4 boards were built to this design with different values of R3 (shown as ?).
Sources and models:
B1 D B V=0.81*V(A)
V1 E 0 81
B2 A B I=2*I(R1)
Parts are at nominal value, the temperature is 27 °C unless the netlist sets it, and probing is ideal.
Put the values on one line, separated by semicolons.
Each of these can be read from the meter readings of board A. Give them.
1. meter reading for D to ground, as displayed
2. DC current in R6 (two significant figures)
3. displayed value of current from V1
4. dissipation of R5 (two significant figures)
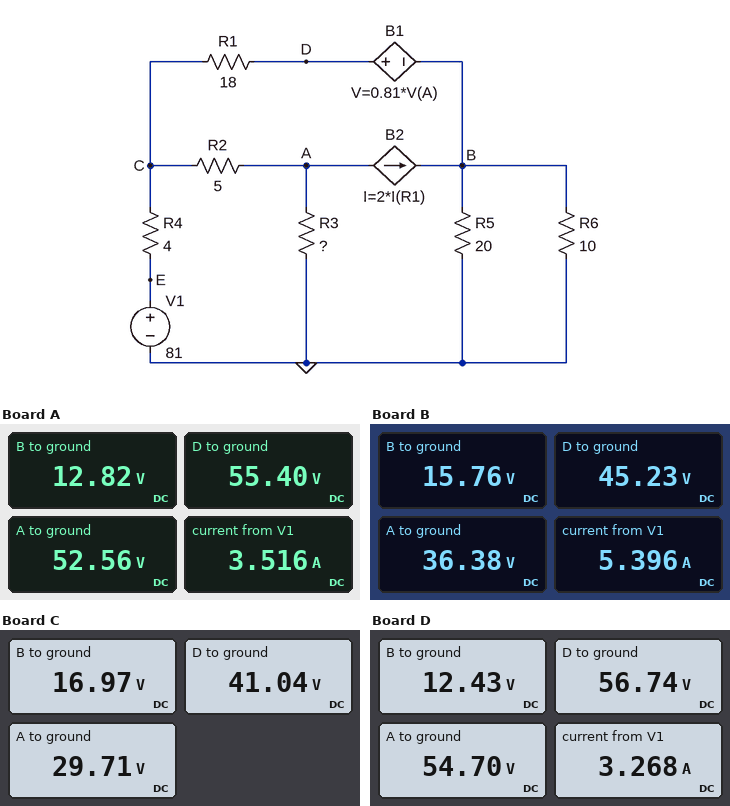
55.40 V; 1.3 A; 3.516 A; 8.2 W
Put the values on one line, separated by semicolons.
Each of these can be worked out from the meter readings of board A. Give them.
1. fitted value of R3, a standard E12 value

33 Ω
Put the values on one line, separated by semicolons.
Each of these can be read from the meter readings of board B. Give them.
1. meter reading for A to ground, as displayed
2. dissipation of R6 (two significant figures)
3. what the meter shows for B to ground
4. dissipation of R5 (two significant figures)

36.38 V; 25 W; 15.76 V; 12 W
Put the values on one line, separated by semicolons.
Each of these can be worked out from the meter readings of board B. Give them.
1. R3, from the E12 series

12 Ω
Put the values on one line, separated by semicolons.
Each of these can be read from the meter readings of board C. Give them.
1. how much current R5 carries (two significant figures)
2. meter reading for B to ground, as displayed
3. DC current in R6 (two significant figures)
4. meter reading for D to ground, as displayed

850 mA; 16.97 V; 1.7 A; 41.04 V
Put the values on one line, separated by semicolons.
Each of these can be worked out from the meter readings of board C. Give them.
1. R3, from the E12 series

8.2 Ω
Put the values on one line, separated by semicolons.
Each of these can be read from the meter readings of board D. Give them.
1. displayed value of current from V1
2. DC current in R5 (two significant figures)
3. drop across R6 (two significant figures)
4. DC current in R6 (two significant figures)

3.268 A; 620 mA; 12 V; 1.2 A
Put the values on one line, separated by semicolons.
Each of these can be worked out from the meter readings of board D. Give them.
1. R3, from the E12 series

39 Ω
